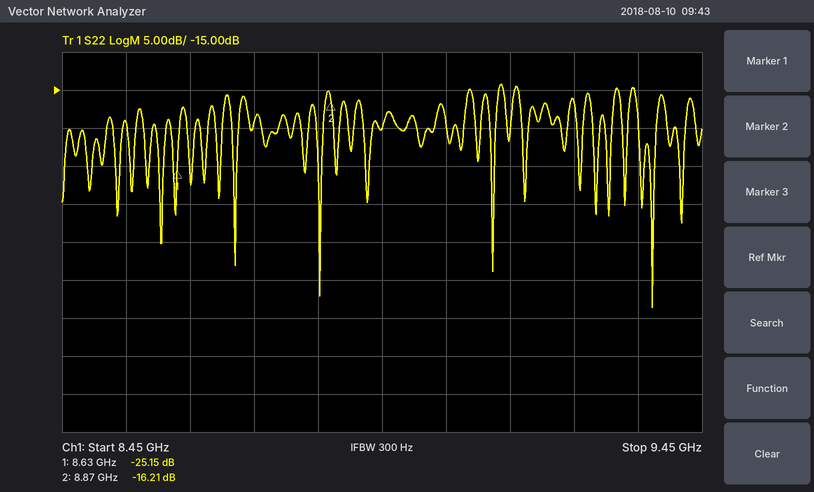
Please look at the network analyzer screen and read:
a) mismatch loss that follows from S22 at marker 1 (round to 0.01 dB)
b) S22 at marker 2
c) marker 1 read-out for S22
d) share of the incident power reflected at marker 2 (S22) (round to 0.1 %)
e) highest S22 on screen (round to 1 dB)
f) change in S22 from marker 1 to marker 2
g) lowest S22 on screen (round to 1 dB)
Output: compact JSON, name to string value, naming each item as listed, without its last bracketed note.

{"mismatch loss that follows from S22 at marker 1": "0.01 dB", "S22 at marker 2": "-16.21 dB", "marker 1 read-out for S22": "-25.15 dB", "share of the incident power reflected at marker 2 (S22)": "2.4 %", "highest S22 on screen": "-14 dB", "change in S22 from marker 1 to marker 2": "8.94 dB", "lowest S22 on screen": "-44 dB"}
